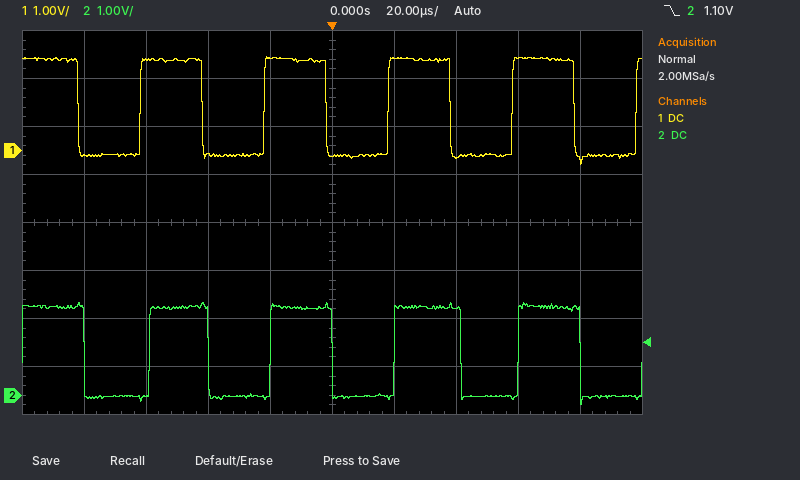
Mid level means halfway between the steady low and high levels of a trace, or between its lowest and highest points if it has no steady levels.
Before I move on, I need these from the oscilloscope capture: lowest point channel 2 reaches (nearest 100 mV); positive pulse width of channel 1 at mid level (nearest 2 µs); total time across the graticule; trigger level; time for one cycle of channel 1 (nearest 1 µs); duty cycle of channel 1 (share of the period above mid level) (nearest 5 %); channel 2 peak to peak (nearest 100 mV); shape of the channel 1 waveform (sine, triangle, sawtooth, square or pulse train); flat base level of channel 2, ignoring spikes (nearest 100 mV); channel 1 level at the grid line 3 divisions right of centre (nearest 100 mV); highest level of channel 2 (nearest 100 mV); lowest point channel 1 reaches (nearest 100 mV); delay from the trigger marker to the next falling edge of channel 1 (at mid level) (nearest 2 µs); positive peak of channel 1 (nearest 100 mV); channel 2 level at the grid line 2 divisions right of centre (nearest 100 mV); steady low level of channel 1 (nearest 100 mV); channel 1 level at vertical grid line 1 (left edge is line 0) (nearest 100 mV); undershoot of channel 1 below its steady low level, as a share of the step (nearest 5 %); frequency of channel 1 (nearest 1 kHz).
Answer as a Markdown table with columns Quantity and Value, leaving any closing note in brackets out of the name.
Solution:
| Quantity | Value |
|---|---|
| lowest point channel 2 reaches | -200 mV |
| positive pulse width of channel 1 at mid level | 20 µs |
| total time across the graticule | 200 µs |
| trigger level | 1.10 V |
| time for one cycle of channel 1 | 40 µs |
| duty cycle of channel 1 (share of the period above mid level) | 50 % |
| channel 2 peak to peak | 2.1 V |
| shape of the channel 1 waveform | square |
| flat base level of channel 2, ignoring spikes | 0.0 V |
| channel 1 level at the grid line 3 divisions right of centre | 1.9 V |
| highest level of channel 2 | 1.9 V |
| lowest point channel 1 reaches | -300 mV |
| delay from the trigger marker to the next falling edge of channel 1 (at mid level) | 38 µs |
| positive peak of channel 1 | 2.0 V |
| channel 2 level at the grid line 2 divisions right of centre | 1.8 V |
| steady low level of channel 1 | -100 mV |
| channel 1 level at vertical grid line 1 (left edge is line 0) | -100 mV |
| undershoot of channel 1 below its steady low level, as a share of the step | 10 % |
| frequency of channel 1 | 25 kHz |
